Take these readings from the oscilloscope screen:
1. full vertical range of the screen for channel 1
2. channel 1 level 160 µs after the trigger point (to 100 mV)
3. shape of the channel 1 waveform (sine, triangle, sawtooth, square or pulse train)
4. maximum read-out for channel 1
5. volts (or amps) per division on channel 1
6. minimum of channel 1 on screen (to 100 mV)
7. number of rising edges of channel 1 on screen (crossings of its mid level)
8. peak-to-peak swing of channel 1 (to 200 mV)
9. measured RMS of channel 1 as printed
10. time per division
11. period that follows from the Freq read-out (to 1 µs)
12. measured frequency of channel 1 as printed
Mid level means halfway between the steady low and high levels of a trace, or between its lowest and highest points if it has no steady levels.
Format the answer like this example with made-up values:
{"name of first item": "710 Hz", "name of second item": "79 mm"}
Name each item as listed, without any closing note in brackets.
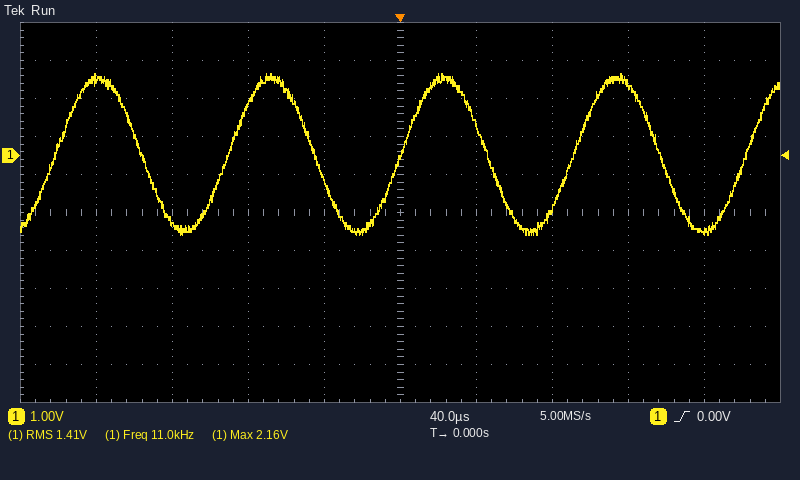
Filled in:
{"full vertical range of the screen for channel 1": "10 V", "channel 1 level 160 µs after the trigger point": "-2.0 V", "shape of the channel 1 waveform": "sine", "maximum read-out for channel 1": "2.16 V", "volts (or amps) per division on channel 1": "1 V", "minimum of channel 1 on screen": "-2.1 V", "number of rising edges of channel 1 on screen": "5", "peak-to-peak swing of channel 1": "4.2 V", "measured RMS of channel 1 as printed": "1.41 V", "time per division": "40 µs", "period that follows from the Freq read-out": "91 µs", "measured frequency of channel 1 as printed": "11.0 kHz"}
